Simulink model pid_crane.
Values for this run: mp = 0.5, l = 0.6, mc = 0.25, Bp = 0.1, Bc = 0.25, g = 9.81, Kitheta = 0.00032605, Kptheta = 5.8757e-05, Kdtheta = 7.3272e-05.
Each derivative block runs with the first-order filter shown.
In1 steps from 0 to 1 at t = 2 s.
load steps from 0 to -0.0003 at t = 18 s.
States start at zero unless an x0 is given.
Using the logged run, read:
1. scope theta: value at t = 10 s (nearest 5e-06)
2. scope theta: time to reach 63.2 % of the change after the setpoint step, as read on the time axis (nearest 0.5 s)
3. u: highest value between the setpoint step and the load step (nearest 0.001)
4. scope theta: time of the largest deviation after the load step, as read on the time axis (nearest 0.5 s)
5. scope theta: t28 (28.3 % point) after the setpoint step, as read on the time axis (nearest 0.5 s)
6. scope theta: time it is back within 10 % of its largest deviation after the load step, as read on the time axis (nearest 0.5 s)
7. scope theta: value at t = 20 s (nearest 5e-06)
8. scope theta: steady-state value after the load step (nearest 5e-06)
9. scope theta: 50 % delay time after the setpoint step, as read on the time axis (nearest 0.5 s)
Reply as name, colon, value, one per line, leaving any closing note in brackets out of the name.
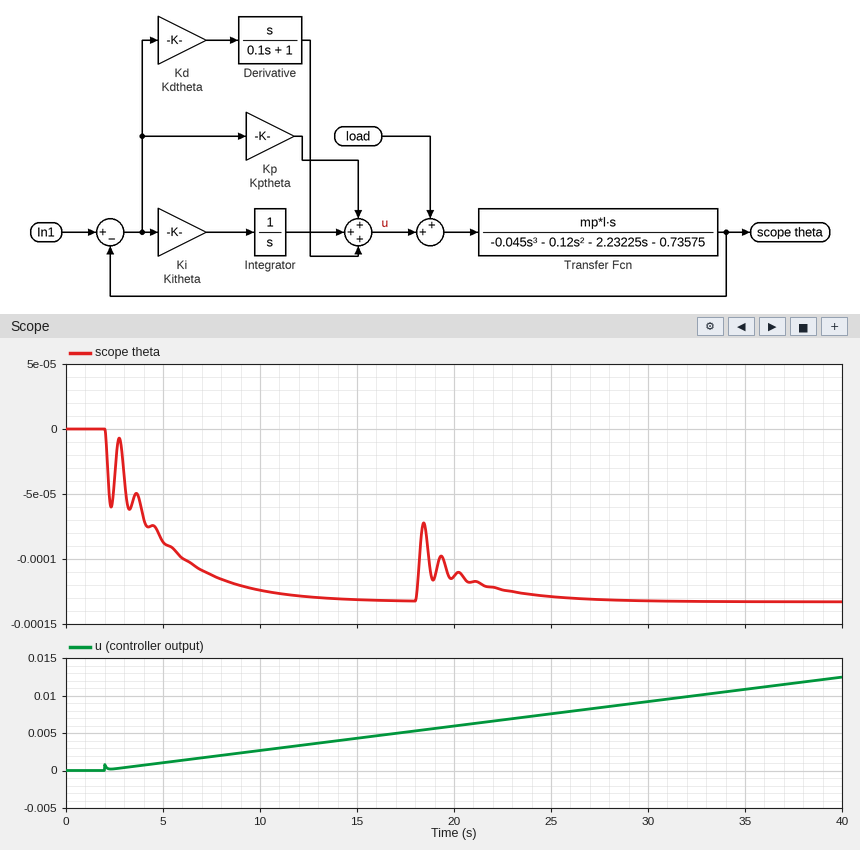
scope theta: value at t = 10 s: -0.000125
scope theta: time to reach 63.2 % of the change after the setpoint step, as read on the time axis: 5.0 s
u: highest value between the setpoint step and the load step: 0.005
scope theta: time of the largest deviation after the load step, as read on the time axis: 18.5 s
scope theta: t28 (28.3 % point) after the setpoint step, as read on the time axis: 2.0 s
scope theta: time it is back within 10 % of its largest deviation after the load step, as read on the time axis: 24.0 s
scope theta: value at t = 20 s: -0.000115
scope theta: steady-state value after the load step: -0.000135
scope theta: 50 % delay time after the setpoint step, as read on the time axis: 4.0 s
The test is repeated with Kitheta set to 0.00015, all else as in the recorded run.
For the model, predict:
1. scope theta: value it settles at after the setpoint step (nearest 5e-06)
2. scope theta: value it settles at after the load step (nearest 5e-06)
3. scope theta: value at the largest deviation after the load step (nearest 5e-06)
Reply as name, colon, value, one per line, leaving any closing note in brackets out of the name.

scope theta: value it settles at after the setpoint step: -0.000060
scope theta: value it settles at after the load step: -0.000060
scope theta: value at the largest deviation after the load step: 0.000000
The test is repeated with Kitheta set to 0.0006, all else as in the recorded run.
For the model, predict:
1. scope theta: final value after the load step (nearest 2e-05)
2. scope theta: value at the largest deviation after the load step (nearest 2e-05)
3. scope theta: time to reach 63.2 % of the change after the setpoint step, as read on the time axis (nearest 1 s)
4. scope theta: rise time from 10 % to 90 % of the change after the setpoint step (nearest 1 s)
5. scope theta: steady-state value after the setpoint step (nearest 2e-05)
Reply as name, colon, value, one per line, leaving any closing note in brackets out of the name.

scope theta: final value after the load step: -0.00024
scope theta: value at the largest deviation after the load step: -0.00018
scope theta: time to reach 63.2 % of the change after the setpoint step, as read on the time axis: 5 s
scope theta: rise time from 10 % to 90 % of the change after the setpoint step: 7 s
scope theta: steady-state value after the setpoint step: -0.00024
